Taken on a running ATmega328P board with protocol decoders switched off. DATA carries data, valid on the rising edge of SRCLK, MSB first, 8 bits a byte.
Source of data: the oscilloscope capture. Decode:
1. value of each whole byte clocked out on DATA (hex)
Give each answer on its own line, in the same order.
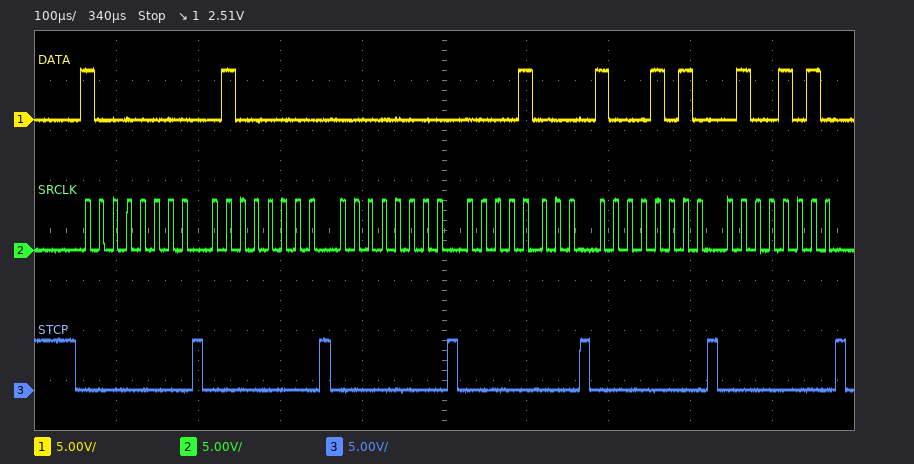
80 40 00 08 8A 4A
